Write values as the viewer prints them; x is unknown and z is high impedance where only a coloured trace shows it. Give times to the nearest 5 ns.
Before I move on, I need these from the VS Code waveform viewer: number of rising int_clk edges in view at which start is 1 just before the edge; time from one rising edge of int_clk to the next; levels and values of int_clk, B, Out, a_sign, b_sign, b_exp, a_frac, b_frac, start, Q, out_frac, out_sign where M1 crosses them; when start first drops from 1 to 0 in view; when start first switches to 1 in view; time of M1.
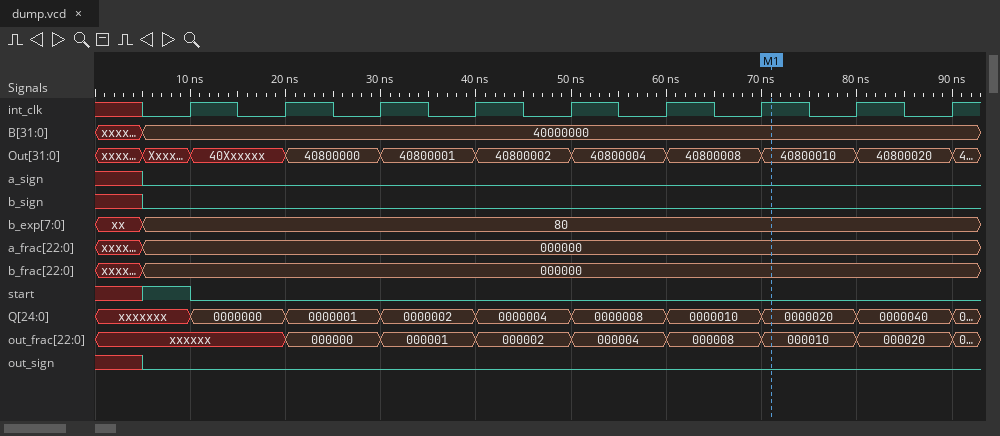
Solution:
1
10 ns
int_clk=1, B=40000000, Out=40800010, a_sign=0, b_sign=0, b_exp=80, a_frac=000000, b_frac=000000, start=0, Q=0000020, out_frac=000010, out_sign=0
10 ns
5 ns
70 ns
